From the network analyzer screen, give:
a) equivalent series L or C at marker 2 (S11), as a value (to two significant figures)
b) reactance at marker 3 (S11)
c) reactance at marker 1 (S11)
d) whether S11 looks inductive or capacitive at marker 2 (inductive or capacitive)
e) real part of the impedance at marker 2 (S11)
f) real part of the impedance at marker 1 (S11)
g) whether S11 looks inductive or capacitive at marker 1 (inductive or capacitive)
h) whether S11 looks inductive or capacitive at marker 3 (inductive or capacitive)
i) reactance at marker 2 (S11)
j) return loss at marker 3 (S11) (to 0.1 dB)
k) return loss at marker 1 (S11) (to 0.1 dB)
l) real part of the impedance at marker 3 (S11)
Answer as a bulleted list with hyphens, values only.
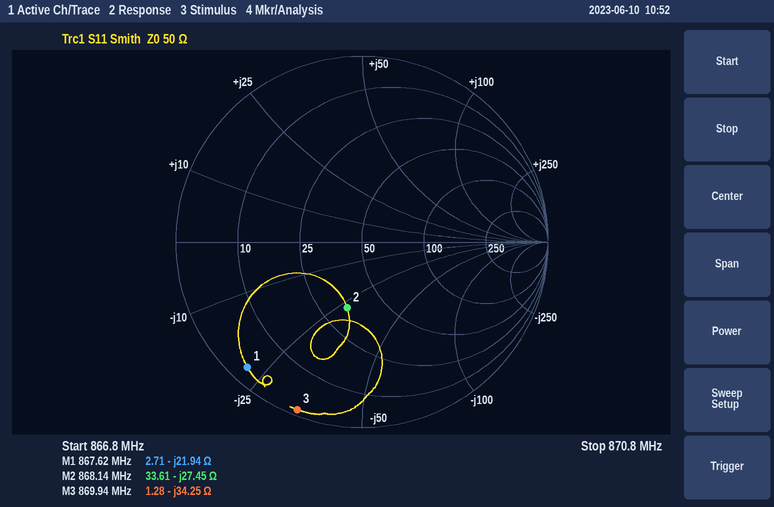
- 6.7 pF
- -34.25 Ω
- -21.94 Ω
- capacitive
- 33.61 Ω
- 2.71 Ω
- capacitive
- capacitive
- -27.45 Ω
- 0.3 dB
- 0.8 dB
- 1.28 Ω
